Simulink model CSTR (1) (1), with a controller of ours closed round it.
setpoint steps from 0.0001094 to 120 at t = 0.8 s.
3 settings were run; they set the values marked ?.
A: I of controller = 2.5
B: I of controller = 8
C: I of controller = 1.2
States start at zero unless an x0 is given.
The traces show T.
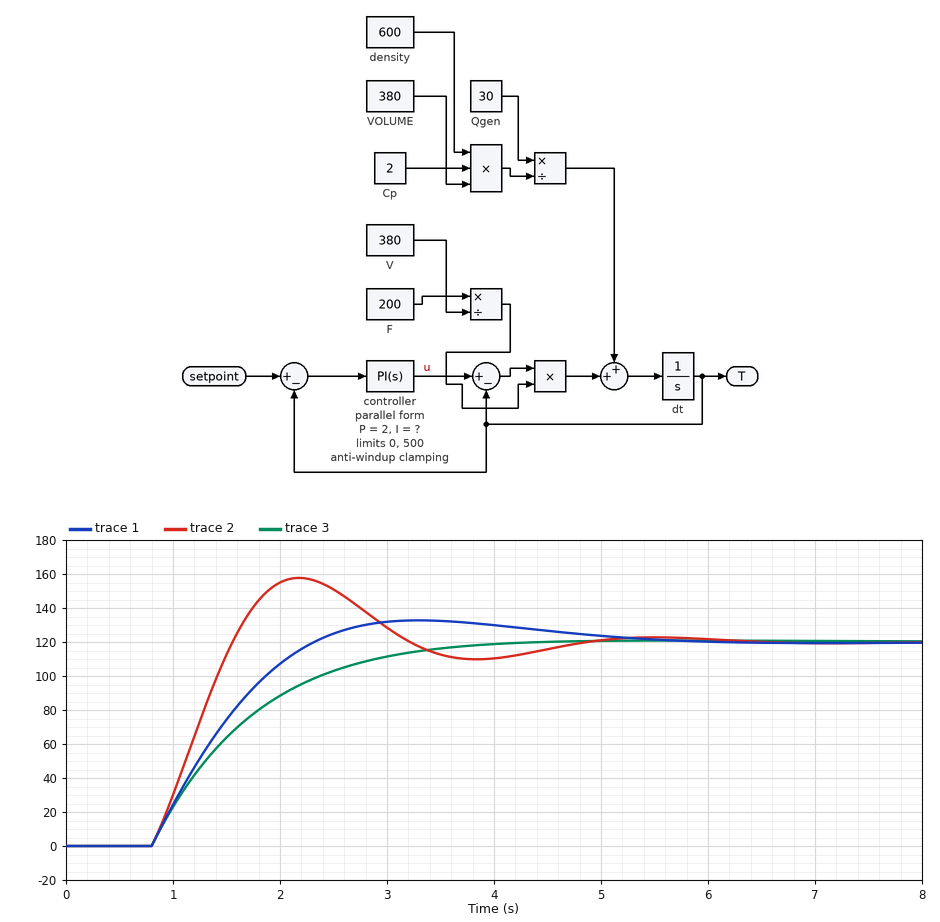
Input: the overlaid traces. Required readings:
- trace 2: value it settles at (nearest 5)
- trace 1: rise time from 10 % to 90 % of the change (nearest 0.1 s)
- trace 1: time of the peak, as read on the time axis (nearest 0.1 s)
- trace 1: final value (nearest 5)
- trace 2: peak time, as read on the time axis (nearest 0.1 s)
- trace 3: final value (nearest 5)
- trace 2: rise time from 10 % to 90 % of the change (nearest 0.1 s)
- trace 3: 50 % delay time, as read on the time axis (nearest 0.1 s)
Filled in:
120
1.1 s
3.3 s
120
2.2 s
120
0.6 s
1.4 s
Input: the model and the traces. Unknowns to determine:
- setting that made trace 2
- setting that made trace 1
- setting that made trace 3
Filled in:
B
A
C
